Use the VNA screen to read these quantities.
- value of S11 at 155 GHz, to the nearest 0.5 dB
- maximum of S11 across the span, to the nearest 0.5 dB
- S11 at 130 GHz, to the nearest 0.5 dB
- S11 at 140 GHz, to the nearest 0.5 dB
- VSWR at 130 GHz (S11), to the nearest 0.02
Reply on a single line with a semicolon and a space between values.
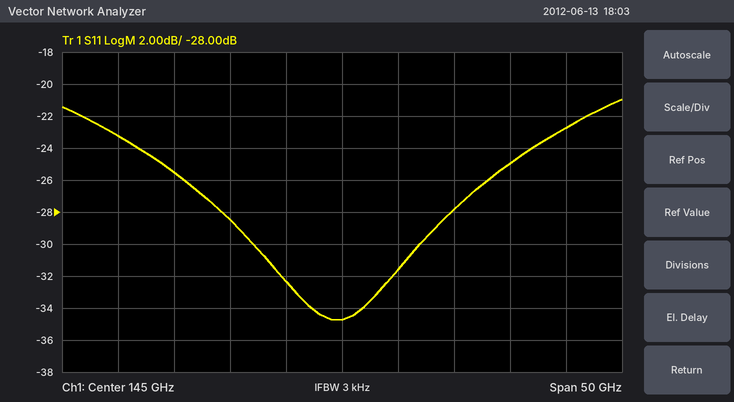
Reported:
-28.0 dB; -21.0 dB; -25.5 dB; -32.5 dB; 1.12
